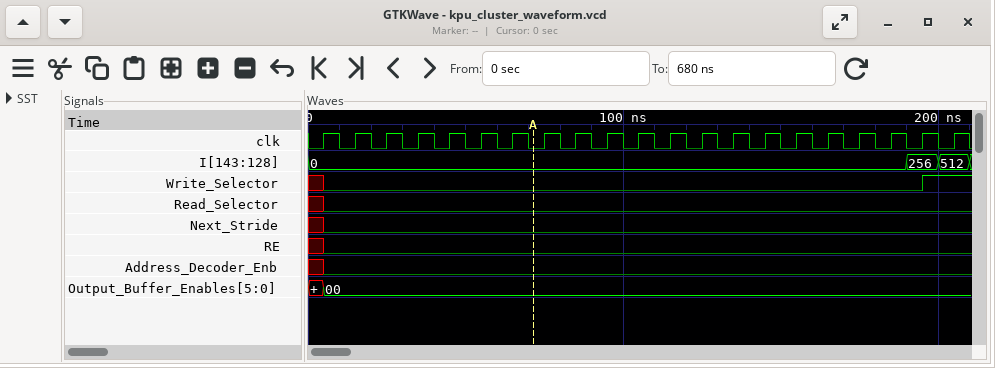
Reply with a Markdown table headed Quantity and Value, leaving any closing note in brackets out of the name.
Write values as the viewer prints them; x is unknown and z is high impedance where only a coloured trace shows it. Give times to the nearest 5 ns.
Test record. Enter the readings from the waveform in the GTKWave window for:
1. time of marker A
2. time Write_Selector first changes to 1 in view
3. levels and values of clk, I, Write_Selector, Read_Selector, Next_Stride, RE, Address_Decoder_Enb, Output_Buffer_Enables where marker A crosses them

| Quantity | Value |
|---|---|
| time of marker A | 70 ns |
| time Write_Selector first changes to 1 in view | 195 ns |
| levels and values of clk, I, Write_Selector, Read_Selector, Next_Stride, RE, Address_Decoder_Enb, Output_Buffer_Enables where marker A crosses them | clk=0, I=0, Write_Selector=0, Read_Selector=0, Next_Stride=0, RE=0, Address_Decoder_Enb=0, Output_Buffer_Enables=00 |
